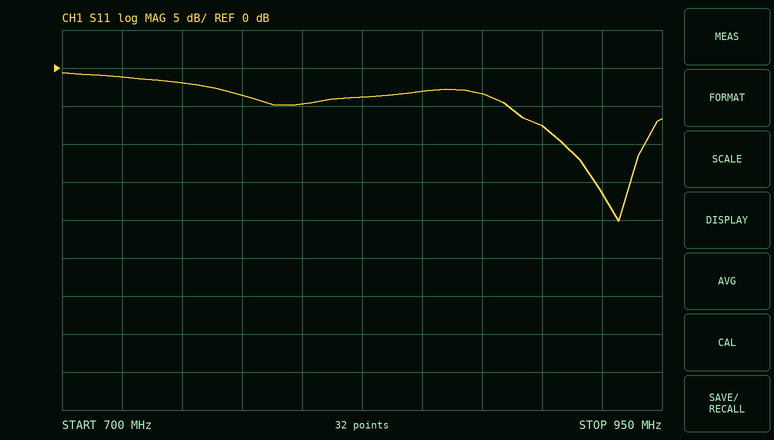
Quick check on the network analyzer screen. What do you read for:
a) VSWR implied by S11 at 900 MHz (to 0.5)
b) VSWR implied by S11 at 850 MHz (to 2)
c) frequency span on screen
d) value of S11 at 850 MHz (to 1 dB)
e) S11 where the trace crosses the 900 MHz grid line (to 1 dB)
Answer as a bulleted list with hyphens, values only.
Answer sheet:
- 2.5
- 6
- 250 MHz
- -3 dB
- -8 dB
